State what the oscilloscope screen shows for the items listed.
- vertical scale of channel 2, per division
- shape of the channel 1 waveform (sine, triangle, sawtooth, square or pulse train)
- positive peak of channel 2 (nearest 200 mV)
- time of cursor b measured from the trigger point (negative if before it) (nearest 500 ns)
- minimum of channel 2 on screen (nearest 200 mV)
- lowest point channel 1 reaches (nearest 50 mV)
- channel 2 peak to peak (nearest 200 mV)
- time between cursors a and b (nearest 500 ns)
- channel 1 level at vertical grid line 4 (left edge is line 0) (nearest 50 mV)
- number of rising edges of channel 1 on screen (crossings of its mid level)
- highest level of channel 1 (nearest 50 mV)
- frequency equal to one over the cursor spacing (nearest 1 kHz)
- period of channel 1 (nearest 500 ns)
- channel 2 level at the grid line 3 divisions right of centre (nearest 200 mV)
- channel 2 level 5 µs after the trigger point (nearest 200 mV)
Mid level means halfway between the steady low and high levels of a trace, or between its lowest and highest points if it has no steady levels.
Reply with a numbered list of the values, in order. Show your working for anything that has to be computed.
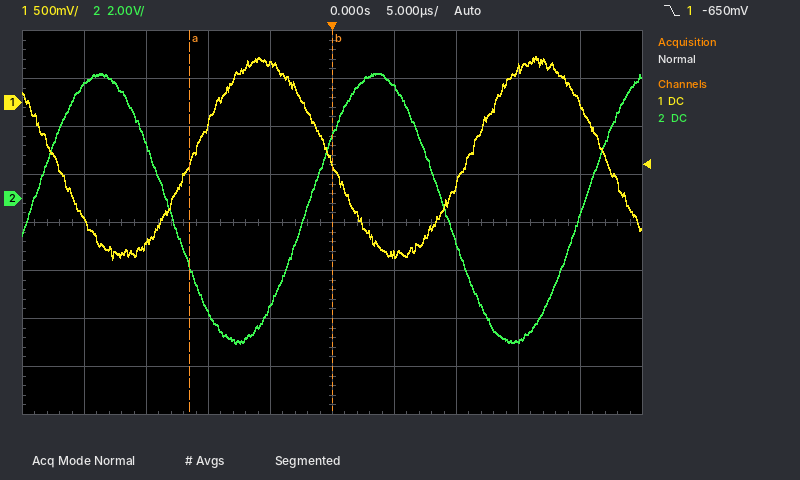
1. 2 V
2. sine
3. 5.2 V
4. 0.0 µs
5. -6.0 V
6. -1.65 V
7. 5.2 V − (-6.0 V) = 11.2 V
8. 11.5 µs
9. 400 mV
10. 2
11. 500 mV
12. 1 / 11.5 µs ≈ 87 kHz
13. 22.0 µs
14. -6.0 V
15. 4.6 V
